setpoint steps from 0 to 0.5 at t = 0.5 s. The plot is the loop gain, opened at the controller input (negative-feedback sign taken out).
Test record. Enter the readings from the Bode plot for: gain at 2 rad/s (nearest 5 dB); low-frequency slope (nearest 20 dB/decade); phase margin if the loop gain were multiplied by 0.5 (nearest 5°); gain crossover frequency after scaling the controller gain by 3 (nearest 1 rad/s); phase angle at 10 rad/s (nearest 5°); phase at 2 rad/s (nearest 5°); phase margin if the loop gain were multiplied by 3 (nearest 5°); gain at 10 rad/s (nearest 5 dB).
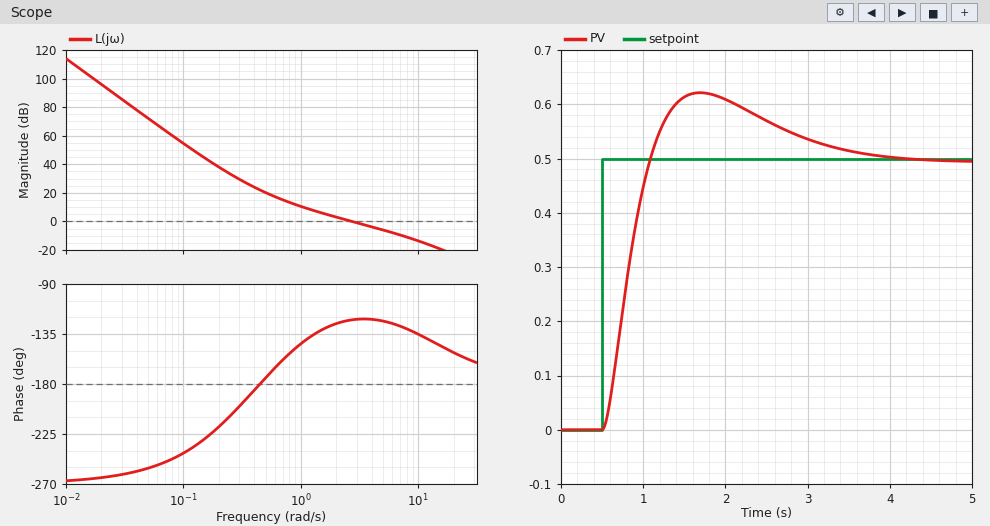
5 dB
-60 dB/decade
50°
7 rad/s
-135°
-125°
50°
-15 dB
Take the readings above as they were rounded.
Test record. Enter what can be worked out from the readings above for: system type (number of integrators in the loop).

3
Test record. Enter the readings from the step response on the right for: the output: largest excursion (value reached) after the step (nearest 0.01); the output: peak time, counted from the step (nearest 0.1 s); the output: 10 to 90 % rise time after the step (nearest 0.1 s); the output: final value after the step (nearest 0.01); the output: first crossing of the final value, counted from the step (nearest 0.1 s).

0.62
1.2 s
0.4 s
0.50
0.6 s
